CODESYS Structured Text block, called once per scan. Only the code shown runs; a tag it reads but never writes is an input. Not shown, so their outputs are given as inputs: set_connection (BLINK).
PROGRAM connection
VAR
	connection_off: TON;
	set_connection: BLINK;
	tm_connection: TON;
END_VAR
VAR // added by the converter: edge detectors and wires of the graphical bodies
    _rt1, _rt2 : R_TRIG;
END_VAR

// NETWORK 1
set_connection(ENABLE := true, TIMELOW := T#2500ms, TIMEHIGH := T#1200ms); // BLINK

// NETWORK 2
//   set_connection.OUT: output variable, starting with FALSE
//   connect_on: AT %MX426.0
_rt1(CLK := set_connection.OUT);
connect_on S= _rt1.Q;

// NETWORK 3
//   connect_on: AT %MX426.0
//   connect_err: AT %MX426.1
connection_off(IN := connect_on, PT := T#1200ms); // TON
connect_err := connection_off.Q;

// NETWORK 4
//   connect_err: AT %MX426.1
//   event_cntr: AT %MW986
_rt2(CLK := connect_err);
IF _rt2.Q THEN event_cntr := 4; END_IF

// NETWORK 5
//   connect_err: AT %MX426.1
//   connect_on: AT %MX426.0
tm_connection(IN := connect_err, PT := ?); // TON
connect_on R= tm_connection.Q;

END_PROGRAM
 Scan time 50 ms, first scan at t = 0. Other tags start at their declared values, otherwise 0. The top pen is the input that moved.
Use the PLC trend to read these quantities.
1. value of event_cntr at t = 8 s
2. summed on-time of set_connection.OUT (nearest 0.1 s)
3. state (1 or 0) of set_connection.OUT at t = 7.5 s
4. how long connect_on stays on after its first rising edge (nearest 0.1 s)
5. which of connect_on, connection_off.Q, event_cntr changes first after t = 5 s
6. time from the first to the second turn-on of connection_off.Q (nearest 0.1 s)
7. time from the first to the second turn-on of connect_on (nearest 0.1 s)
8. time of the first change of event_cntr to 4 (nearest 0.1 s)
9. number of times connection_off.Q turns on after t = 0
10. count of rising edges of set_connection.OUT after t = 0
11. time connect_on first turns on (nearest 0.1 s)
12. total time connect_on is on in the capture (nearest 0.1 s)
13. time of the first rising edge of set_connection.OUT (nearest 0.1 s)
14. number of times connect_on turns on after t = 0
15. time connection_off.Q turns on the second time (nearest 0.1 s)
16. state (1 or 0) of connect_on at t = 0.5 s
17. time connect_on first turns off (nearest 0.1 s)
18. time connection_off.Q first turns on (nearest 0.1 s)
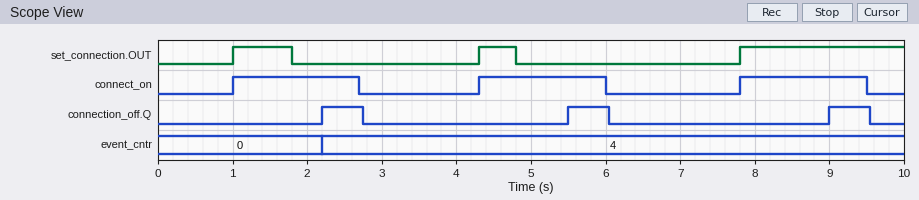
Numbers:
4
3.5 s
0
1.7 s
connection_off.Q
3.3 s
3.3 s
2.2 s
3
3
1.0 s
5.1 s
1.0 s
3
5.5 s
0
2.7 s
2.2 s
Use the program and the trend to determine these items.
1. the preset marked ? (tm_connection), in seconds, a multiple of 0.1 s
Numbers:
0.5 s
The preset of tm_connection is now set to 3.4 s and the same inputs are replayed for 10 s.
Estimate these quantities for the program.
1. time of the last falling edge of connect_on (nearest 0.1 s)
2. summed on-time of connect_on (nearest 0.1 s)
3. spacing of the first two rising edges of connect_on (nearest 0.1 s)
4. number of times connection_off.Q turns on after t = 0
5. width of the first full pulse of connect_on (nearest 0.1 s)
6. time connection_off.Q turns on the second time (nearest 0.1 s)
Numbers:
5.6 s
6.8 s
6.8 s
2
4.6 s
9.0 s
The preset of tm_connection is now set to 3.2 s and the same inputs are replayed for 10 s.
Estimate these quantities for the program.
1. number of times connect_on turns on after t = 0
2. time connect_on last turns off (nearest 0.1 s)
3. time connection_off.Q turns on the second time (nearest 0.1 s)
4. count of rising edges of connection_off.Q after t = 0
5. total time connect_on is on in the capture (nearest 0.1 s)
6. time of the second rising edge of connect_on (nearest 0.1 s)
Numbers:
2
5.4 s
9.0 s
2
6.6 s
7.8 s
